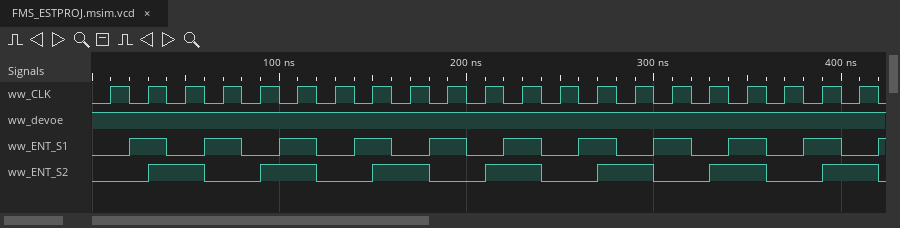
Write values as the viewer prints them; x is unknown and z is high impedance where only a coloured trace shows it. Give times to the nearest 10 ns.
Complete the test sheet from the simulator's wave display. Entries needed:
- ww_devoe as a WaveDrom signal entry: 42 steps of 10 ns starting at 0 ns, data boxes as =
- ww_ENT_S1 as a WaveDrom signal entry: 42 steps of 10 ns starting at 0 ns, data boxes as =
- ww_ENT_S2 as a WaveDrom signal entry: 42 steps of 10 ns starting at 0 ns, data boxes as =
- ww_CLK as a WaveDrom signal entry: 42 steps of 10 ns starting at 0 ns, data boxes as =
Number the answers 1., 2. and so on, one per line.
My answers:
1. {name: 'ww_devoe', wave: '1.........................................'}
2. {name: 'ww_ENT_S1', wave: '0.1.0.1.0.1.0.1.0.1.0.1.0.1.0.1.0.1.0.1.0.'}
3. {name: 'ww_ENT_S2', wave: '0..1..0..1..0..1..0..1..0..1..0..1..0..1..'}
4. {name: 'ww_CLK', wave: '010101010101010101010101010101010101010101'}
